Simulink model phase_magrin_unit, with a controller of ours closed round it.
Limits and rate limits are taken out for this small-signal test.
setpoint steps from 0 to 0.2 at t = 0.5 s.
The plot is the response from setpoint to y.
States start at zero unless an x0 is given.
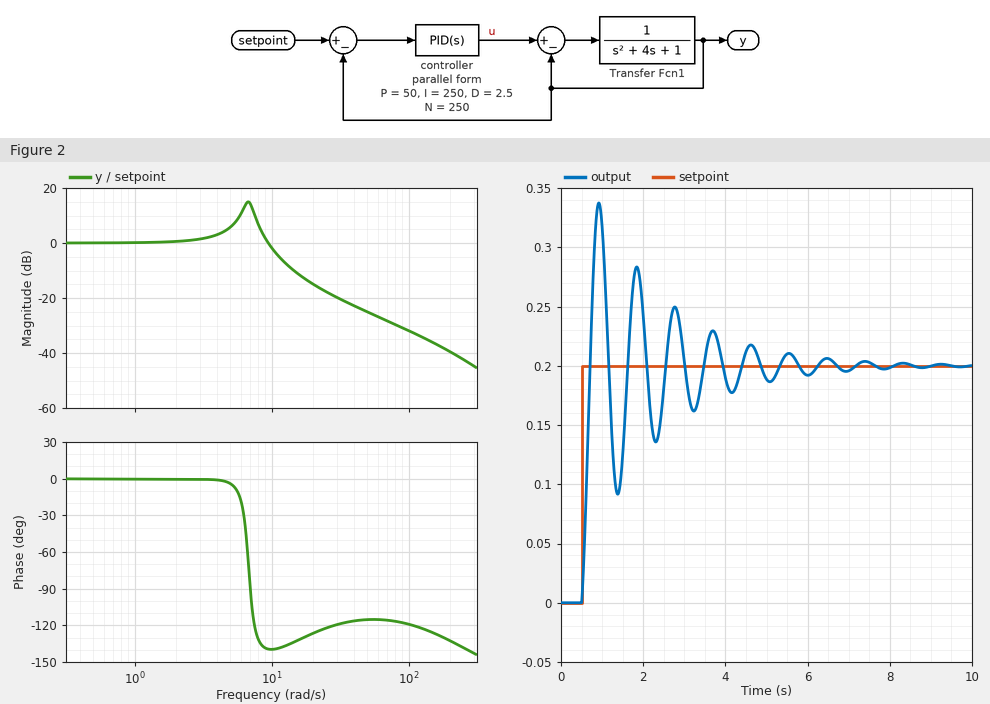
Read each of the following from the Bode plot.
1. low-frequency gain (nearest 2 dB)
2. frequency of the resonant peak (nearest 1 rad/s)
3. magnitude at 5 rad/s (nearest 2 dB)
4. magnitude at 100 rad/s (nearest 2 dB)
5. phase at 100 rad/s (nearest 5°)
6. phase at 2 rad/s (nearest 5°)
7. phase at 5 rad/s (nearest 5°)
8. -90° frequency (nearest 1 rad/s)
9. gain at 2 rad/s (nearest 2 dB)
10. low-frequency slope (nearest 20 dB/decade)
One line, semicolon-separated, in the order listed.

0 dB; 7 rad/s; 6 dB; -32 dB; -120°; 0°; -5°; 7 rad/s; 0 dB; 0 dB/decade
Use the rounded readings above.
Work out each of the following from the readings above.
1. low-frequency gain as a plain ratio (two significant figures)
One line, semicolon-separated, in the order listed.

1.0
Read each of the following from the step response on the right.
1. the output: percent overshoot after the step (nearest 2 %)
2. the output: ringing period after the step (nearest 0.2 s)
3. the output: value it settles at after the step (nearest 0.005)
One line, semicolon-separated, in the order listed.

68 %; 1.0 s; 0.200
